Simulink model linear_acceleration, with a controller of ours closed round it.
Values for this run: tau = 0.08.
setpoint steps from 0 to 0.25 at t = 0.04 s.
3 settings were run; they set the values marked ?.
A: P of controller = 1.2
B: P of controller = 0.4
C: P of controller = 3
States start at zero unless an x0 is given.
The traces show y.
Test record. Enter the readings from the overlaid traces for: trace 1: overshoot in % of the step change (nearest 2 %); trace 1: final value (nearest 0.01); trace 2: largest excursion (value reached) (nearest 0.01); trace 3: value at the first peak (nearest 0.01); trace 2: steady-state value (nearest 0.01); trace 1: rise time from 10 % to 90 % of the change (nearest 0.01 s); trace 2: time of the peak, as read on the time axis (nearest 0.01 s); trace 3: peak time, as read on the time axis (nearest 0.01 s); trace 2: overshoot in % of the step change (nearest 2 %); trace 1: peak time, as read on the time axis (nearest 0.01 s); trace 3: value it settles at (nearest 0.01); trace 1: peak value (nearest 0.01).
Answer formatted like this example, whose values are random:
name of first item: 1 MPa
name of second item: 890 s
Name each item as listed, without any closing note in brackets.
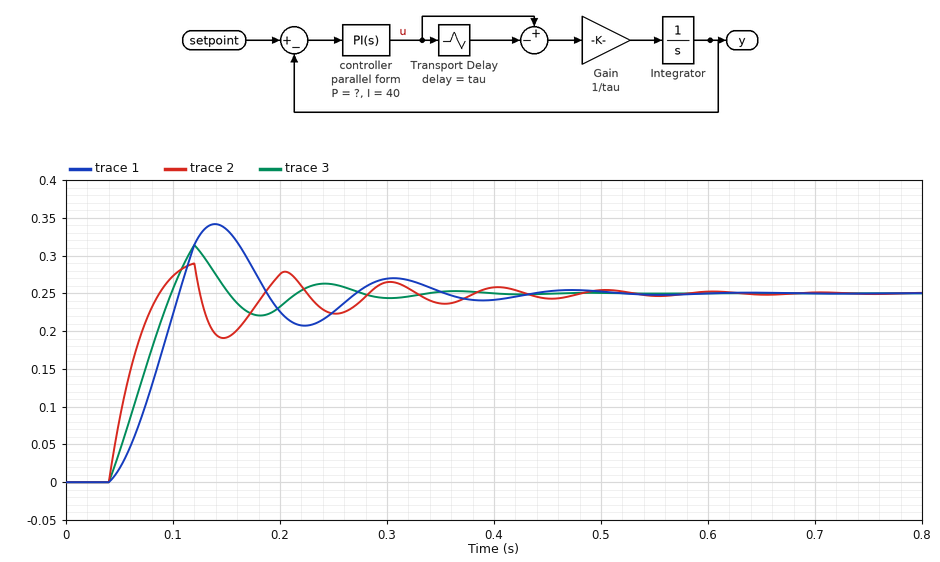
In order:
trace 1: overshoot in % of the step change: 36 %
trace 1: final value: 0.25
trace 2: largest excursion (value reached): 0.29
trace 3: value at the first peak: 0.31
trace 2: steady-state value: 0.25
trace 1: rise time from 10 % to 90 % of the change: 0.05 s
trace 2: time of the peak, as read on the time axis: 0.12 s
trace 3: peak time, as read on the time axis: 0.12 s
trace 2: overshoot in % of the step change: 16 %
trace 1: peak time, as read on the time axis: 0.14 s
trace 3: value it settles at: 0.25
trace 1: peak value: 0.34
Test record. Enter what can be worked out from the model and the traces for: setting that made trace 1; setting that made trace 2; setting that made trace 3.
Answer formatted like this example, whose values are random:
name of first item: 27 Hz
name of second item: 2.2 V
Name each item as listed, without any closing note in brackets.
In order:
setting that made trace 1: B
setting that made trace 2: C
setting that made trace 3: A
